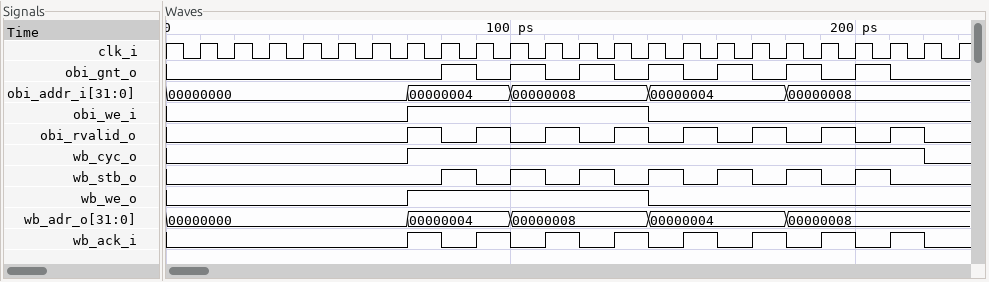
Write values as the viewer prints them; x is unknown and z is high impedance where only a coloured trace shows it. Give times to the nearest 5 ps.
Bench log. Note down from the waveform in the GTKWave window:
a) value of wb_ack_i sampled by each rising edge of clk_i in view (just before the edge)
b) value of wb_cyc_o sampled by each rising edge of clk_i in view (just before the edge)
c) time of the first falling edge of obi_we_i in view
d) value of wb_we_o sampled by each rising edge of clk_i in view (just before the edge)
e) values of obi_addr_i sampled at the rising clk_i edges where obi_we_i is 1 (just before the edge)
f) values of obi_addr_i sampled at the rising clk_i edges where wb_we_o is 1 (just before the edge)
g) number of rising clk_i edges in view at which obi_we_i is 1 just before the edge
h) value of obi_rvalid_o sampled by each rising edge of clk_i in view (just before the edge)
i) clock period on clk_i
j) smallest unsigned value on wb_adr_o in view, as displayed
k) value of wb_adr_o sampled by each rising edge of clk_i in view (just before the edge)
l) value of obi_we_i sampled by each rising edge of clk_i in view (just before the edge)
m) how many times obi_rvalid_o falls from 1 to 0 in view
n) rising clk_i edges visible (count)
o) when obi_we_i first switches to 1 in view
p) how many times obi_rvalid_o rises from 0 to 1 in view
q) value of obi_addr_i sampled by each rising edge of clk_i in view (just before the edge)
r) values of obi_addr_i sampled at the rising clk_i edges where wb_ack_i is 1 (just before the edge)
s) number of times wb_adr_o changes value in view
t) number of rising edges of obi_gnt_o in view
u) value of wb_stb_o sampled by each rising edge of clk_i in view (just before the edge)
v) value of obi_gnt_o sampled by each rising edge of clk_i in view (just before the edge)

0 0 0 0 0 0 0 1 0 1 0 1 0 1 0 1 0 1 0 1 0 1 0
0 0 0 0 0 0 0 1 1 1 1 1 1 1 1 1 1 1 1 1 1 1 0
140 ps
0 0 0 0 0 0 0 1 1 1 1 1 1 1 0 0 0 0 0 0 0 0 0
00000004, 00000004, 00000004, 00000008, 00000008, 00000008, 00000008
00000004, 00000004, 00000004, 00000008, 00000008, 00000008, 00000008
7
0 0 0 0 0 0 0 1 0 1 0 1 0 1 0 1 0 1 0 1 0 1 0
10 ps
00000000
00000000, 00000000, 00000000, 00000000, 00000000, 00000000, 00000000, 00000004, 00000004, 00000004, 00000008, 00000008, 00000008, 00000008, 00000004, 00000004, 00000004, 00000004, 00000008, 00000008, 00000008, 00000008, 00000008
0 0 0 0 0 0 0 1 1 1 1 1 1 1 0 0 0 0 0 0 0 0 0
8
23
70 ps
8
00000000, 00000000, 00000000, 00000000, 00000000, 00000000, 00000000, 00000004, 00000004, 00000004, 00000008, 00000008, 00000008, 00000008, 00000004, 00000004, 00000004, 00000004, 00000008, 00000008, 00000008, 00000008, 00000008
00000004, 00000004, 00000008, 00000008, 00000004, 00000004, 00000008, 00000008
4
7
0 0 0 0 0 0 0 0 1 0 1 0 1 0 1 0 1 0 1 0 1 0 0
0 0 0 0 0 0 0 0 1 0 1 0 1 0 1 0 1 0 1 0 1 0 0
